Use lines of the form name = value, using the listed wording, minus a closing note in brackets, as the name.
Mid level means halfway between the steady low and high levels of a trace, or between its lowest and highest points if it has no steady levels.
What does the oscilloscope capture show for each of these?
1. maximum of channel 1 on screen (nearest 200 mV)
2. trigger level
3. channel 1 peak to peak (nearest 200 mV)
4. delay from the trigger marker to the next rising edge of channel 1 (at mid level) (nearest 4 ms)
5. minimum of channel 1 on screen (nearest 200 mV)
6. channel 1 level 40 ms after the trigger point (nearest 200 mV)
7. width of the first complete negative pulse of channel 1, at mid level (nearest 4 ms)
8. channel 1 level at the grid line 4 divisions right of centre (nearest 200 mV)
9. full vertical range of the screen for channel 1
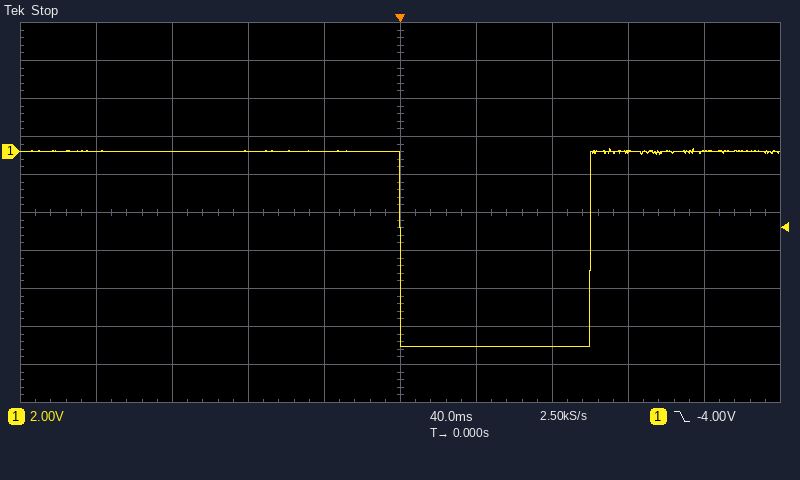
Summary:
maximum of channel 1 on screen = 200 mV
trigger level = -4.00 V
channel 1 peak to peak = 10.4 V
delay from the trigger marker to the next rising edge of channel 1 (at mid level) = 100 ms
minimum of channel 1 on screen = -10.2 V
channel 1 level 40 ms after the trigger point = -10.2 V
width of the first complete negative pulse of channel 1, at mid level = 100 ms
channel 1 level at the grid line 4 divisions right of centre = 0.0 V
full vertical range of the screen for channel 1 = 20 V
